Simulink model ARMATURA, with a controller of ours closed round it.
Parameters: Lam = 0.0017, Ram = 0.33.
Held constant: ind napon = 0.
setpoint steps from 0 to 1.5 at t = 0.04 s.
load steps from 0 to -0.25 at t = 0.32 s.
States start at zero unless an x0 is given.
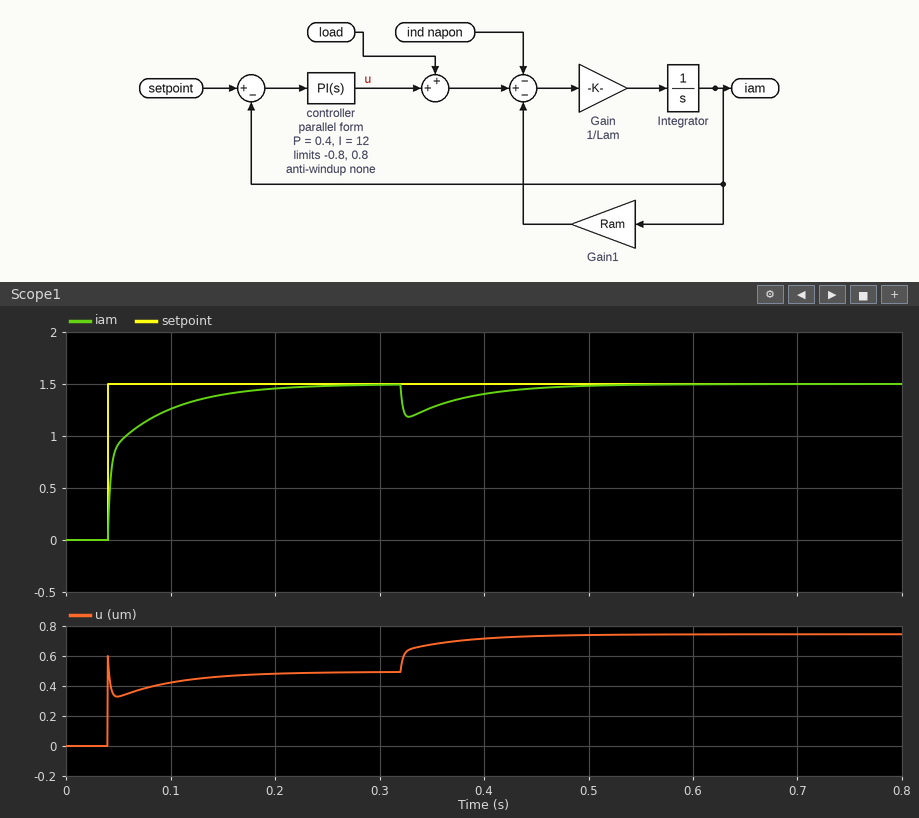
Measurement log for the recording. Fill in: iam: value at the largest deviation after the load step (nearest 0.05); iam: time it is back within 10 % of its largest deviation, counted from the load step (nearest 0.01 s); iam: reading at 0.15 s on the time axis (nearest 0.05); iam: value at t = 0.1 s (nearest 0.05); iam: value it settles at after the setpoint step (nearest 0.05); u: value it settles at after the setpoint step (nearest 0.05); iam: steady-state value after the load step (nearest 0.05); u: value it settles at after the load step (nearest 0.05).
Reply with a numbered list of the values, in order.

1. 1.20
2. 0.15 s
3. 1.40
4. 1.25
5. 1.50
6. 0.50
7. 1.50
8. 0.75
